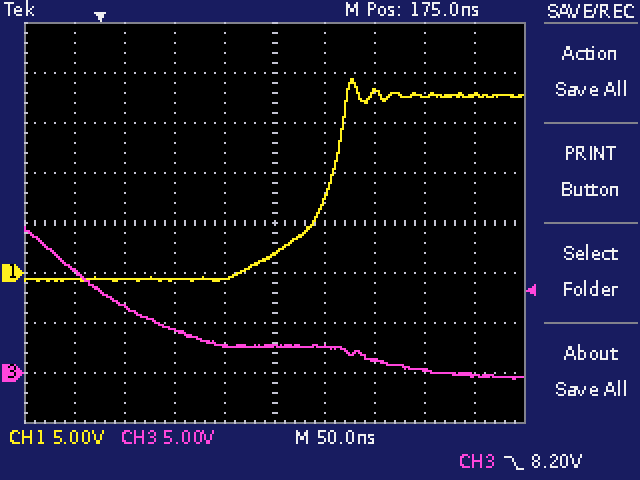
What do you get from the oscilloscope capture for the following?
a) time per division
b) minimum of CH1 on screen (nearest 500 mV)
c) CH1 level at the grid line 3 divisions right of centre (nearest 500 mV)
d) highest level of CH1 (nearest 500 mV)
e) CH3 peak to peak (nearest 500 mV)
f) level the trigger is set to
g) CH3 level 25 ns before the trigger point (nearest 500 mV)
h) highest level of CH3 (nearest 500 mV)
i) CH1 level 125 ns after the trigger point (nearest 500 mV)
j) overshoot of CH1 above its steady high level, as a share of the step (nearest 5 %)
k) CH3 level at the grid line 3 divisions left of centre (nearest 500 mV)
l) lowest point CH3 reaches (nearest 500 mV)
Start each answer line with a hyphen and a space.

- 50 ns
- -1.0 V
- 17.5 V
- 19.5 V
- 15.0 V
- 8.20 V
- 10.0 V
- 14.5 V
- -500 mV
- 10 %
- 6.5 V
- -500 mV
